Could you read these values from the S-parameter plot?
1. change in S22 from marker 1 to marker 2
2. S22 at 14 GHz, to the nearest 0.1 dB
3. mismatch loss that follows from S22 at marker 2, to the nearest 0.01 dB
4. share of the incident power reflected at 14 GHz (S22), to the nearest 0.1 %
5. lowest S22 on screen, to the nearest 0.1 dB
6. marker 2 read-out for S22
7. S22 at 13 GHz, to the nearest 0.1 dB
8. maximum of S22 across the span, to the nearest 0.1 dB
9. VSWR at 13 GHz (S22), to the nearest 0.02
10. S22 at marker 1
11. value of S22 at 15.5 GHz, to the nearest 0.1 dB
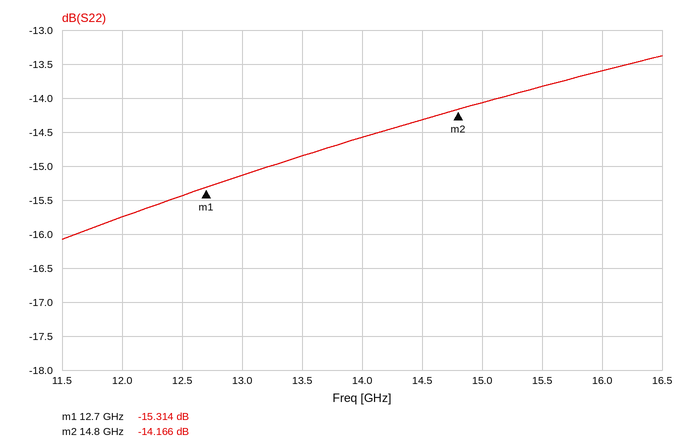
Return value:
1.148 dB
-14.6 dB
0.17 dB
3.5 %
-16.1 dB
-14.166 dB
-15.1 dB
-13.4 dB
1.42
-15.314 dB
-13.8 dB
